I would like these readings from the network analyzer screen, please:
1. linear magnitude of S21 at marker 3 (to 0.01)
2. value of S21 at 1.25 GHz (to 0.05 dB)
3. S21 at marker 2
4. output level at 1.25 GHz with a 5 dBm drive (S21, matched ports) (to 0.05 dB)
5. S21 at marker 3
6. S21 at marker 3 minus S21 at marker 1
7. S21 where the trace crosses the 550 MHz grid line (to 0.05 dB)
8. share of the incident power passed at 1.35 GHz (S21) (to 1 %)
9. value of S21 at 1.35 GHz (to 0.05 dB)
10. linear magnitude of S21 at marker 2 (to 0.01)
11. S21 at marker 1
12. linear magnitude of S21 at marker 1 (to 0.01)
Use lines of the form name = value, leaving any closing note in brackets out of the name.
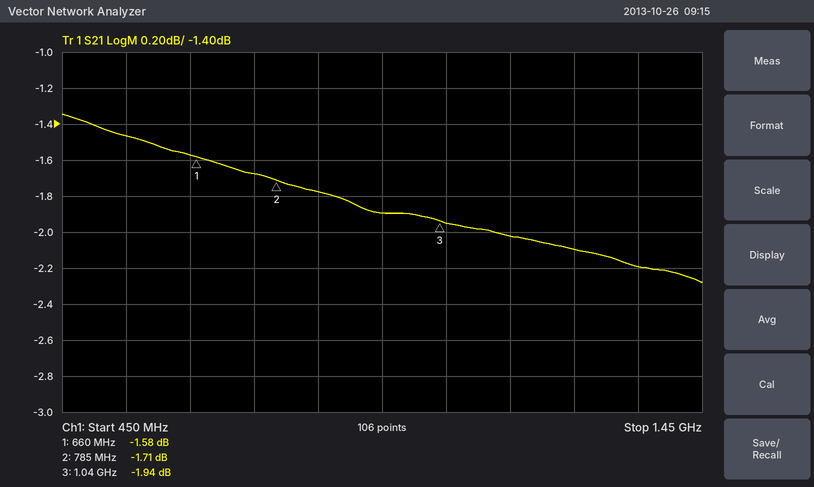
linear magnitude of S21 at marker 3 = 0.80
value of S21 at 1.25 GHz = -2.10 dB
S21 at marker 2 = -1.71 dB
output level at 1.25 GHz with a 5 dBm drive (S21, matched ports) = 2.90 dBm
S21 at marker 3 = -1.94 dB
S21 at marker 3 minus S21 at marker 1 = -0.36 dB
S21 where the trace crosses the 550 MHz grid line = -1.45 dB
share of the incident power passed at 1.35 GHz (S21) = 60 %
value of S21 at 1.35 GHz = -2.20 dB
linear magnitude of S21 at marker 2 = 0.82
S21 at marker 1 = -1.58 dB
linear magnitude of S21 at marker 1 = 0.83
